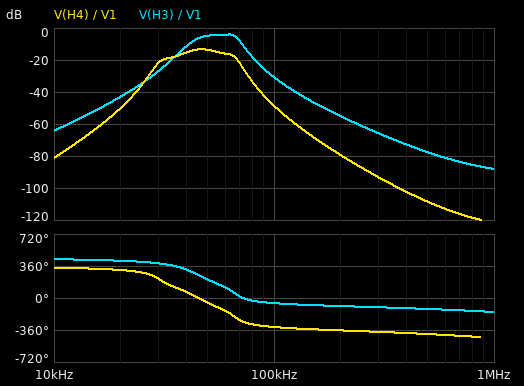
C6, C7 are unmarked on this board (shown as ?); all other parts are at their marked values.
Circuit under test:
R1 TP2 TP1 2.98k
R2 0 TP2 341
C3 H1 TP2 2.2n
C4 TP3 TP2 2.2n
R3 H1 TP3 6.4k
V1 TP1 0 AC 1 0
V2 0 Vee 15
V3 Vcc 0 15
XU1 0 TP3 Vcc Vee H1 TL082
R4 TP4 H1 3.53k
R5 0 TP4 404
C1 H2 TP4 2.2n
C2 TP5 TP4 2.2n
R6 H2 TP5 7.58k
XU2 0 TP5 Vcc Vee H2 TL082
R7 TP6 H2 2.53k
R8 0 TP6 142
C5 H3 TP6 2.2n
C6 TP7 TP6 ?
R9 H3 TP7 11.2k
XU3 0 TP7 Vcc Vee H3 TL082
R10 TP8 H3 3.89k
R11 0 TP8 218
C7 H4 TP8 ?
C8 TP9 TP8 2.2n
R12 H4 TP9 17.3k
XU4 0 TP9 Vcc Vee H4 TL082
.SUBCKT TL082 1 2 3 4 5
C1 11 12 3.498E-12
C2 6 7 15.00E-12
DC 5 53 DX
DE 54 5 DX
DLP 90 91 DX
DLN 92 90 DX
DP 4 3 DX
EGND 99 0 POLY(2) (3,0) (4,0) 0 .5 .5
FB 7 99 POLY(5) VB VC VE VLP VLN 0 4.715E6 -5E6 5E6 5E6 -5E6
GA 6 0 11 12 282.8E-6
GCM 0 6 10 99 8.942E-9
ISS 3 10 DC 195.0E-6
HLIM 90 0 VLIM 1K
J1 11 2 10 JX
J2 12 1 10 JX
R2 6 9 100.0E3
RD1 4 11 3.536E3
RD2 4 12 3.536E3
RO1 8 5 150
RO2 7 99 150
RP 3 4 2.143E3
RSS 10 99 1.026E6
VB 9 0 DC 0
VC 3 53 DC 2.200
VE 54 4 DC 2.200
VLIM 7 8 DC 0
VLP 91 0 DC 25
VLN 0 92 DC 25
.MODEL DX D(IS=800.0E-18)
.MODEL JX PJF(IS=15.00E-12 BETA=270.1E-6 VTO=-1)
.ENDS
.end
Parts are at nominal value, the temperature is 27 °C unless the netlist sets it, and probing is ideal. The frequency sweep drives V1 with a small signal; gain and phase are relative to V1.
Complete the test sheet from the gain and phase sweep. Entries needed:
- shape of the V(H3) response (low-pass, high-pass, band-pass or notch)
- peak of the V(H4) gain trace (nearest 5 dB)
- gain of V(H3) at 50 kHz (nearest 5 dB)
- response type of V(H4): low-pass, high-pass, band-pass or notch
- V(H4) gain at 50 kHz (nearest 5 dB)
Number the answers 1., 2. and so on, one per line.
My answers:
1. band-pass
2. -15 dB
3. -5 dB
4. band-pass
5. -15 dB
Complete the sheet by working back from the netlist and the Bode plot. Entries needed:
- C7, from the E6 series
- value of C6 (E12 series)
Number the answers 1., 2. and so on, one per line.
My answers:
1. 3.3 nF
2. 1.5 nF
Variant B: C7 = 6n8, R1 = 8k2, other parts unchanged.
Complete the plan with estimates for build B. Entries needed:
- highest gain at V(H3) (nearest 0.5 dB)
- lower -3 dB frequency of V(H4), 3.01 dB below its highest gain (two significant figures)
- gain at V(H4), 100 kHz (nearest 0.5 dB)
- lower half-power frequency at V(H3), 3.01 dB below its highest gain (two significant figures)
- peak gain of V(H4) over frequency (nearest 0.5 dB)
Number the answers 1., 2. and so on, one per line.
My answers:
1. -13.5 dB
2. 40 kHz
3. -64.0 dB
4. 43 kHz
5. -30.5 dB
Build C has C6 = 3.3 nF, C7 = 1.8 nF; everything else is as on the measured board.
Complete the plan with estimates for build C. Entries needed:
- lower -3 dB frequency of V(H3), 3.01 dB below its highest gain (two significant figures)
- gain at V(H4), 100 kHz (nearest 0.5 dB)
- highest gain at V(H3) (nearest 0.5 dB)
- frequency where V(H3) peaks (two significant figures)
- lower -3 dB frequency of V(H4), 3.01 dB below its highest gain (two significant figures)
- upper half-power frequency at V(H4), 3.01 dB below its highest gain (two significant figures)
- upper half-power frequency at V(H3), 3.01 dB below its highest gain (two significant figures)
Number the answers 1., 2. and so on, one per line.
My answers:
1. 42 kHz
2. -46.0 dB
3. 9.0 dB
4. 45 kHz
5. 40 kHz
6. 47 kHz
7. 49 kHz
